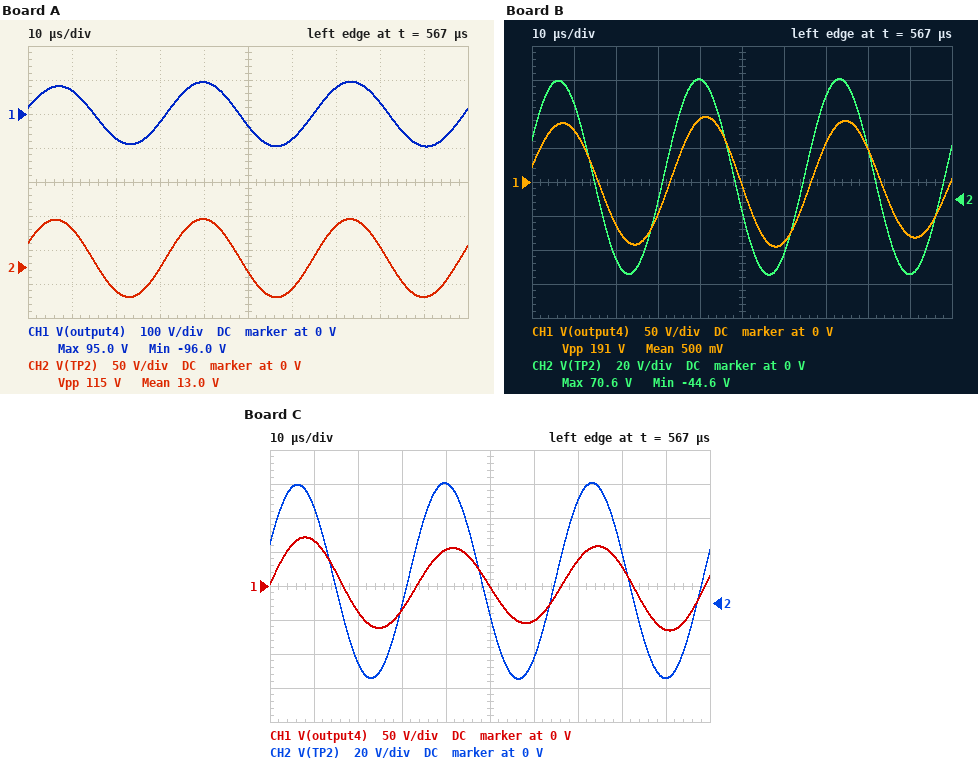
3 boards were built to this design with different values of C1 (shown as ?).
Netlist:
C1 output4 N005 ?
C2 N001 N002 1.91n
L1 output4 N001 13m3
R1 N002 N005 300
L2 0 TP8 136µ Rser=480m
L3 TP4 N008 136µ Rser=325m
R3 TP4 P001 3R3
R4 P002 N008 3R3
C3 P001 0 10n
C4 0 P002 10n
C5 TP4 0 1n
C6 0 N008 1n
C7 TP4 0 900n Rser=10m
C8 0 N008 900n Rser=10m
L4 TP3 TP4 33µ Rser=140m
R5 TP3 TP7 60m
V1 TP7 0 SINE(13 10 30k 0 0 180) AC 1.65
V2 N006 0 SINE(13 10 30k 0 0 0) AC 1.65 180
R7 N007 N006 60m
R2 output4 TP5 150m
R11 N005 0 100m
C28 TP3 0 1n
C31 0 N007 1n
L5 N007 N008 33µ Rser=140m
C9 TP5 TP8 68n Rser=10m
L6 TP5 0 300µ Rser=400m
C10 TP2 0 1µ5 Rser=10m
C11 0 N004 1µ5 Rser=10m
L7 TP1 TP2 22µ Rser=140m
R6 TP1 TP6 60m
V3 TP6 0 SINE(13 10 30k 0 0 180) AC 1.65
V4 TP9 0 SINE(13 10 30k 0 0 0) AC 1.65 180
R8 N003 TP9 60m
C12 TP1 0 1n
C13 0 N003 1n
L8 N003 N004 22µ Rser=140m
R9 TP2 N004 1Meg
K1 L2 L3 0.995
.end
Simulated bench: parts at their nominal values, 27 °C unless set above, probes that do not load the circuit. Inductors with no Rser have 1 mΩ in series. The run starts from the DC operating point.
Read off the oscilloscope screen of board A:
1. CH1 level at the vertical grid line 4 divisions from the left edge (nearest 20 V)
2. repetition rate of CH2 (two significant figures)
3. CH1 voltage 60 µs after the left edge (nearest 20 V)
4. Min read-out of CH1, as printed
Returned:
100 V
30 kHz
-80 V
-96.0 V
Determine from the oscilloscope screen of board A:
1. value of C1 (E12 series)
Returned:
33 nF
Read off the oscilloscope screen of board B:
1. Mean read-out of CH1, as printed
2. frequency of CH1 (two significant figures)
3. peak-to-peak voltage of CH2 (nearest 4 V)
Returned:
500 mV
30 kHz
116 V
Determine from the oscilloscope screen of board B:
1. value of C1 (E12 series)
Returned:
39 nF
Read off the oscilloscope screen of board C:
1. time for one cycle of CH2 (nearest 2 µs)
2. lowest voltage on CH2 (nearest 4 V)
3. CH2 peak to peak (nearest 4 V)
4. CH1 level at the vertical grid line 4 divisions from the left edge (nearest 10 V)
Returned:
34 µs
-44 V
116 V
50 V
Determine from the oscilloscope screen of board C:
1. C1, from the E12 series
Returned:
47 nF
